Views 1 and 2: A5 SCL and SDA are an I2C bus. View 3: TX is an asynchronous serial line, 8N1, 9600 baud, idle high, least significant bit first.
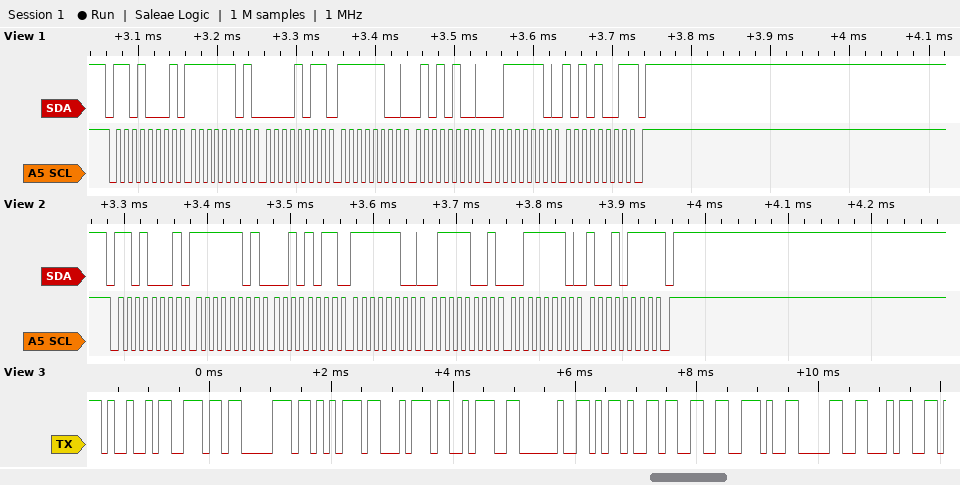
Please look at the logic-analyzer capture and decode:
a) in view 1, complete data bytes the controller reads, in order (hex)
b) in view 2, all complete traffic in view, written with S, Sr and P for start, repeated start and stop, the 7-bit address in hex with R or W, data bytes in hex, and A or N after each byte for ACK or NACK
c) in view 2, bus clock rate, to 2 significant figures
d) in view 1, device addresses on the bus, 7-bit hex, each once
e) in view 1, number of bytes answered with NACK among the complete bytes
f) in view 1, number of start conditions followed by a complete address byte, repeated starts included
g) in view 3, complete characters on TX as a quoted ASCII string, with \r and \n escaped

FD 0B FC 54 3E A9
S 68R A FD A 2B A FC A 79 A 3E A 97 N P
100 kHz
0x68
1
1
"Input: -3.04"
